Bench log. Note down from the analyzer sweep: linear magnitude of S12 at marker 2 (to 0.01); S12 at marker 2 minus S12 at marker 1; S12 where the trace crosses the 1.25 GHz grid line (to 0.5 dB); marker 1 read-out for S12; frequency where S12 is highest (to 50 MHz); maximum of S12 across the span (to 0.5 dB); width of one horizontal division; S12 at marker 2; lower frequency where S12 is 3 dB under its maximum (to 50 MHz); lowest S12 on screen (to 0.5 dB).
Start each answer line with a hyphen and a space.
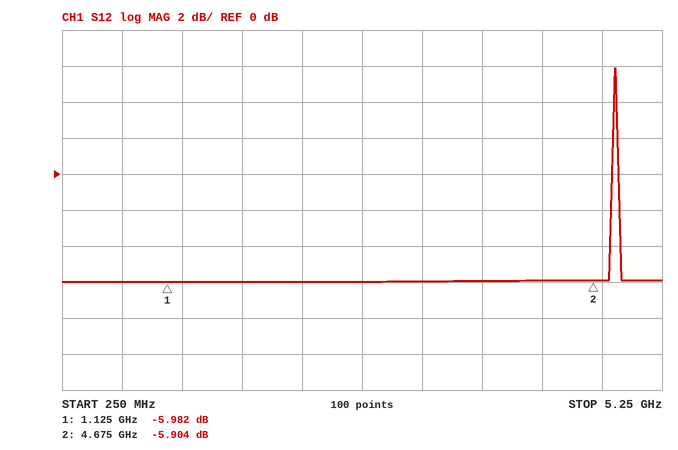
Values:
- 0.51
- 0.078 dB
- -6.0 dB
- -5.982 dB
- 4.85 GHz
- 6.0 dB
- 500 MHz
- -5.904 dB
- 4.85 GHz
- -6.0 dB
